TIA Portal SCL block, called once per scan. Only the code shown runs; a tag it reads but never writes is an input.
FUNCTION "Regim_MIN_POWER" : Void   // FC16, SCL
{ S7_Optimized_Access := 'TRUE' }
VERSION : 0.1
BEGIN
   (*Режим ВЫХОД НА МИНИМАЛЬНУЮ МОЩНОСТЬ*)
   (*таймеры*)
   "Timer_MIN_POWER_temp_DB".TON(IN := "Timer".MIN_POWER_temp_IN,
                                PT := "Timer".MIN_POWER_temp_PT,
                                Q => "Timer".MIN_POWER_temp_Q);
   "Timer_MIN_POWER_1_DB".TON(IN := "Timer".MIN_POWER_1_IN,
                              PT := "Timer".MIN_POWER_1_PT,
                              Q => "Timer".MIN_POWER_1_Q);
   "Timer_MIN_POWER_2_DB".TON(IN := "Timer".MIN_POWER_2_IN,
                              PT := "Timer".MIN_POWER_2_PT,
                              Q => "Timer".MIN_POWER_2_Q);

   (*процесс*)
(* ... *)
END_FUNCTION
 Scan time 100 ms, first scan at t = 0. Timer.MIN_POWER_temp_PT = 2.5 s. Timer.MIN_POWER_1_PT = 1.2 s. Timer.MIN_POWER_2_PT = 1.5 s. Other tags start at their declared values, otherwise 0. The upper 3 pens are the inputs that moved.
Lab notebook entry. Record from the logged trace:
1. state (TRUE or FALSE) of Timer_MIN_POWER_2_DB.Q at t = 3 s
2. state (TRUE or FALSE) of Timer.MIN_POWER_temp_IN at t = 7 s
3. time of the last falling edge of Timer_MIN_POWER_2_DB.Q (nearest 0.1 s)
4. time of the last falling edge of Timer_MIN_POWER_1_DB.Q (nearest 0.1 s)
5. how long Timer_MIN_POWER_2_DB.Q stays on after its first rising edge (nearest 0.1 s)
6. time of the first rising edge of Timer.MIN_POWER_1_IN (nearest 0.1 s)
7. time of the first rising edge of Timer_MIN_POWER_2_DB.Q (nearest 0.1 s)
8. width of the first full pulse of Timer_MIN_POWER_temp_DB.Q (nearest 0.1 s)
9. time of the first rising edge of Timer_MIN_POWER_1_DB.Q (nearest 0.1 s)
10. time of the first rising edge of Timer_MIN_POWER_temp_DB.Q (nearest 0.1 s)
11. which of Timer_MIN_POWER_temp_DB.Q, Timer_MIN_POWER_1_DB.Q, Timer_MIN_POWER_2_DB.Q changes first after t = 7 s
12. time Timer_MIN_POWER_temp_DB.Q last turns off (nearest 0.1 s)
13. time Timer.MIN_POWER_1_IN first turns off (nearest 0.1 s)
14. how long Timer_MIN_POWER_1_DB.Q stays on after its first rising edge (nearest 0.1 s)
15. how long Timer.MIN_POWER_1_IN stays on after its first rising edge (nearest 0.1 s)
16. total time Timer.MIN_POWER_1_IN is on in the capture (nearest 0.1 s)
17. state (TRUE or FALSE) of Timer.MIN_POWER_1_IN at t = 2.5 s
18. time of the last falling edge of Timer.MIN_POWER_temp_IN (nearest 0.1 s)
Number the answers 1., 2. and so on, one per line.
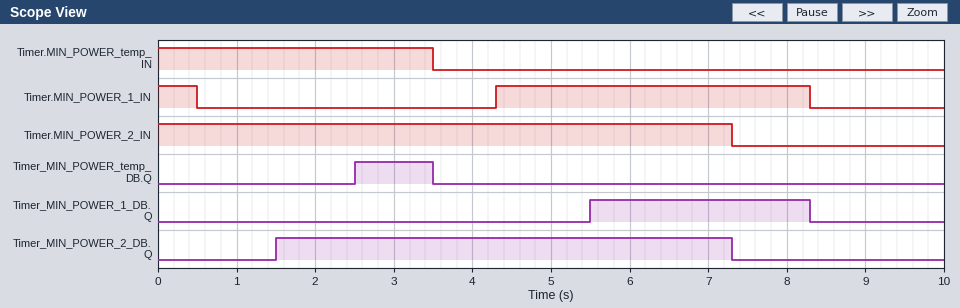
1. TRUE
2. FALSE
3. 7.3 s
4. 8.3 s
5. 5.8 s
6. 4.3 s
7. 1.5 s
8. 1.0 s
9. 5.5 s
10. 2.5 s
11. Timer_MIN_POWER_2_DB.Q
12. 3.5 s
13. 0.5 s
14. 2.8 s
15. 4.0 s
16. 4.5 s
17. FALSE
18. 3.5 s
